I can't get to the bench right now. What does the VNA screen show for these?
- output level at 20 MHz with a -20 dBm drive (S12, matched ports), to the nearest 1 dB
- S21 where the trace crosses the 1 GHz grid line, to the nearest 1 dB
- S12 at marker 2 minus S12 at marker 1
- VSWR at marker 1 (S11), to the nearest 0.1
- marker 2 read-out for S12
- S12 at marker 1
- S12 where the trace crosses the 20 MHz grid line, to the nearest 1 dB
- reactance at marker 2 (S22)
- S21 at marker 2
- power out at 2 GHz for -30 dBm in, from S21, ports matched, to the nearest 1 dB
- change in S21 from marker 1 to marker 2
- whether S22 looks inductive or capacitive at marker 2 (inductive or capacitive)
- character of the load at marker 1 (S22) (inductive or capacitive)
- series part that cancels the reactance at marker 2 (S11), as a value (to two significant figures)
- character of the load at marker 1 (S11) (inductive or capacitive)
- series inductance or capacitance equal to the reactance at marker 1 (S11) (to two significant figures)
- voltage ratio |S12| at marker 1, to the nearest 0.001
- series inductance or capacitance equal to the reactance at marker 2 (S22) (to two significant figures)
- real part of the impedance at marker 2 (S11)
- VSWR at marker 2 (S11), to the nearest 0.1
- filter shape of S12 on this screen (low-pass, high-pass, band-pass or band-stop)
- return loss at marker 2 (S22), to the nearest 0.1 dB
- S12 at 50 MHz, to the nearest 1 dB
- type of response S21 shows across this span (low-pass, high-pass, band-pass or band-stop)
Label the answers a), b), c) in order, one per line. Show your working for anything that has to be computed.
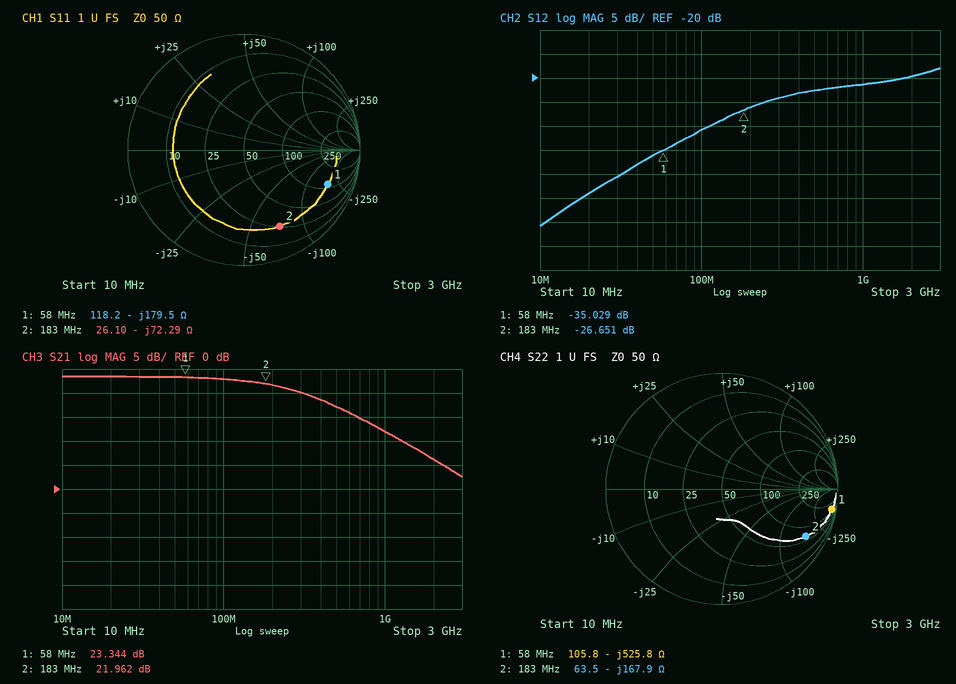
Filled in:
a) -20 dBm + (-44 dB) = -64 dBm
b) 12 dB
c) -26.651 − (-35.029) = 8.378 dB
d) 8.1
e) -26.651 dB
f) -35.029 dB
g) -44 dB
h) -167.9 Ω
i) 21.962 dB
j) -30 dBm + (6 dB) = -24 dBm
k) 21.962 − (23.344) = -1.382 dB
l) capacitive
m) capacitive
n) L = 72.29 Ω/(2π × 183 MHz) ≈ 63 nH
o) capacitive
p) C = 1/(2π × 58 MHz × 179.5 Ω) ≈ 15 pF
q) 10^(-35.029/20) ≈ 0.018
r) C = 1/(2π × 183 MHz × 167.9 Ω) ≈ 5.2 pF
s) 26.10 Ω
t) 6.3
u) high-pass
v) 1.6 dB
w) -36 dB
x) low-pass
